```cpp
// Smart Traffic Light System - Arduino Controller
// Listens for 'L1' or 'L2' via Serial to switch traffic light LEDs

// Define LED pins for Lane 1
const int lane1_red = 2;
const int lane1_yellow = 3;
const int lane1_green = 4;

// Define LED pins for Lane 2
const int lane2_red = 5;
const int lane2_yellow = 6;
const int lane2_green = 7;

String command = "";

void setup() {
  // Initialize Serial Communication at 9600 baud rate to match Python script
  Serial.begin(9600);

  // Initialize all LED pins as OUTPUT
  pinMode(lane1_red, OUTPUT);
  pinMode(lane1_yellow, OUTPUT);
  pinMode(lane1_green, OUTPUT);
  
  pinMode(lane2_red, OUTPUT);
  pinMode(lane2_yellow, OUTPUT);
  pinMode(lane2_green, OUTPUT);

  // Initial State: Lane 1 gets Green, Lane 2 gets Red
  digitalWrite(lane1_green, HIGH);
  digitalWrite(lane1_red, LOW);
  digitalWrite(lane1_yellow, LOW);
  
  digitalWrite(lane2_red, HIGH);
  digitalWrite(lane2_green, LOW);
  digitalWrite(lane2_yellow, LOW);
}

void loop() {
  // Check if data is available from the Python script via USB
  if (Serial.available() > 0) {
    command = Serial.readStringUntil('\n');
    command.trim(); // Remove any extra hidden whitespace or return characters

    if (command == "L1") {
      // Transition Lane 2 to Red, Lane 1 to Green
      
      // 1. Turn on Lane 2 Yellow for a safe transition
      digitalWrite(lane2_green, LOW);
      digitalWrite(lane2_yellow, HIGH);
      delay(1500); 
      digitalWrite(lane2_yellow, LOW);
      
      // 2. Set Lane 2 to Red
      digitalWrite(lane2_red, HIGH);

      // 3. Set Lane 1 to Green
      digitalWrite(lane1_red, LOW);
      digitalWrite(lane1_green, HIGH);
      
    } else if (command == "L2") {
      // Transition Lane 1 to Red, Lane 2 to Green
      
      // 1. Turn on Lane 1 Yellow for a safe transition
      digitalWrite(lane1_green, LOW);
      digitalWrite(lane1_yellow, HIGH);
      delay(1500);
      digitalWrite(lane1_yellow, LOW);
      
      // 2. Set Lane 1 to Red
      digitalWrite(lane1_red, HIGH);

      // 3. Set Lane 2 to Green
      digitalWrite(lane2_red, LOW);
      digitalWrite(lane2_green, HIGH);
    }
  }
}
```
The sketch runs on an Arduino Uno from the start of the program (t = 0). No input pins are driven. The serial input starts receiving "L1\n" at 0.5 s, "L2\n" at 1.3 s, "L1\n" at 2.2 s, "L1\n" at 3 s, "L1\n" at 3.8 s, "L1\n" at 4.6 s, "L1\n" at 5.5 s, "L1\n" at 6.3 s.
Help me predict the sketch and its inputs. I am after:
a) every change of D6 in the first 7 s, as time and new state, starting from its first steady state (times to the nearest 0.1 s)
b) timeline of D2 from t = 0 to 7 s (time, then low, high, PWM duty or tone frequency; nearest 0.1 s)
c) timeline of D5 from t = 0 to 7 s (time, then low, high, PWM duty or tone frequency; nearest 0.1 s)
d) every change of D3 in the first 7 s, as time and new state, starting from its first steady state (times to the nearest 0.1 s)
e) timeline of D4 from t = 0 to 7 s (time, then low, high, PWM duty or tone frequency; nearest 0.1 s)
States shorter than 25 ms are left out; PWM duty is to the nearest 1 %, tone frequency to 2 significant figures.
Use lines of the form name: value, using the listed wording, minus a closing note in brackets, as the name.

every change of D6 in the first 7 s, as time and new state, starting from its first steady state: 0 s low; 0.5 s high; 2 s low; 3.5 s high
timeline of D2 from t = 0 to 7 s: 0 s low; 3.5 s high; 5 s low
timeline of D5 from t = 0 to 7 s: 0 s high; 3.5 s low; 5 s high
every change of D3 in the first 7 s, as time and new state, starting from its first steady state: 0 s low; 2 s high; 3.5 s low
timeline of D4 from t = 0 to 7 s: 0 s high; 2 s low; 5 s high
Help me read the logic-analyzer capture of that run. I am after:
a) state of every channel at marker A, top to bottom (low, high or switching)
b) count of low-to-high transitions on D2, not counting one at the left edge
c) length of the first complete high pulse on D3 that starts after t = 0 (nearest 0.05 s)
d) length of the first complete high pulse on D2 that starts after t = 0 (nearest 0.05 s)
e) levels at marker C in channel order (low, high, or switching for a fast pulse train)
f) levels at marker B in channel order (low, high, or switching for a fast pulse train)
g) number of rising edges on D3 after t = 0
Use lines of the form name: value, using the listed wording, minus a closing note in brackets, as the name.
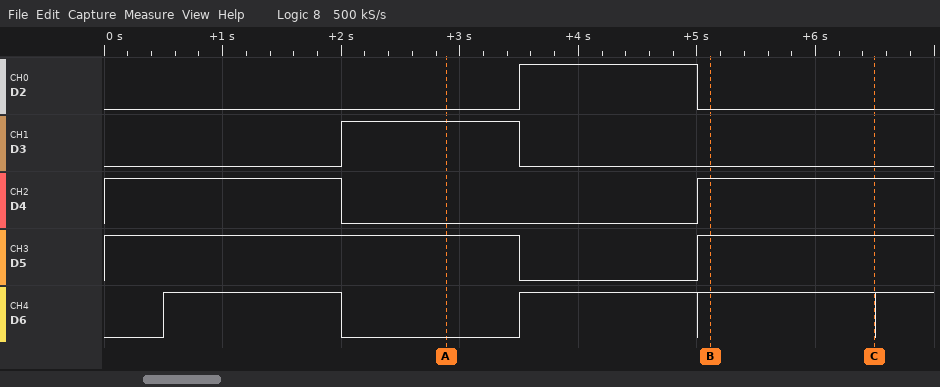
state of every channel at marker A, top to bottom: D2 low, D3 high, D4 low, D5 high, D6 low
count of low-to-high transitions on D2, not counting one at the left edge: 1
length of the first complete high pulse on D3 that starts after t = 0: 1.50 s
length of the first complete high pulse on D2 that starts after t = 0: 1.50 s
levels at marker C in channel order: D2 low, D3 low, D4 high, D5 high, D6 high
levels at marker B in channel order: D2 low, D3 low, D4 high, D5 high, D6 high
number of rising edges on D3 after t = 0: 1
